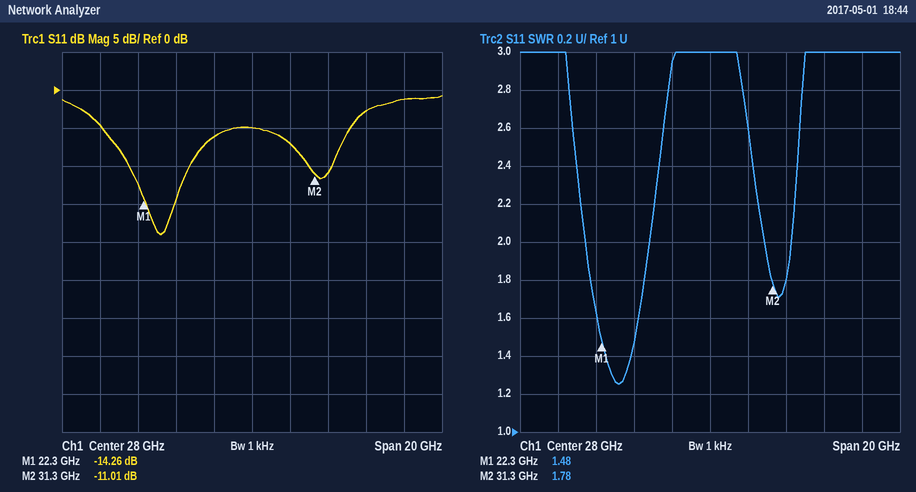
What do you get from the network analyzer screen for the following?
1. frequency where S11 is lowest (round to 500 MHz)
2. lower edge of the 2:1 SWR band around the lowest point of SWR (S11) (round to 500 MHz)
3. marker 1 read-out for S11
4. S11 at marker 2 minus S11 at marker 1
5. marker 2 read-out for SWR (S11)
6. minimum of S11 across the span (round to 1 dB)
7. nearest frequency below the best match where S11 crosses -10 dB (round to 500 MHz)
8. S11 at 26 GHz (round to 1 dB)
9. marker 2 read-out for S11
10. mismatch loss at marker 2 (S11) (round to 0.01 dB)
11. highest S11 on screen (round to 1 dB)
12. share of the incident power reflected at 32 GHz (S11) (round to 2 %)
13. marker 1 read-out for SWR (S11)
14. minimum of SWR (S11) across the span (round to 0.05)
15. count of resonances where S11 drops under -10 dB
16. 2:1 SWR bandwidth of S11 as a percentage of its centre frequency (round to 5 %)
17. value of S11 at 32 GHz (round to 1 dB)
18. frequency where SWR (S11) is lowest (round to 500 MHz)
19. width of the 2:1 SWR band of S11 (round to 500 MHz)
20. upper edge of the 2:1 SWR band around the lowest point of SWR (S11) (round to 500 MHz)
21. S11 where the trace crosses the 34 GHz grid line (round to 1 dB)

23.0 GHz
21.5 GHz
-14.26 dB
3.25 dB
1.78
-19 dB
21.5 GHz
-6 dB
-11.01 dB
0.36 dB
-1 dB
8 %
1.48
1.25
2
15 %
-11 dB
23.0 GHz
3.5 GHz
25.0 GHz
-3 dB
